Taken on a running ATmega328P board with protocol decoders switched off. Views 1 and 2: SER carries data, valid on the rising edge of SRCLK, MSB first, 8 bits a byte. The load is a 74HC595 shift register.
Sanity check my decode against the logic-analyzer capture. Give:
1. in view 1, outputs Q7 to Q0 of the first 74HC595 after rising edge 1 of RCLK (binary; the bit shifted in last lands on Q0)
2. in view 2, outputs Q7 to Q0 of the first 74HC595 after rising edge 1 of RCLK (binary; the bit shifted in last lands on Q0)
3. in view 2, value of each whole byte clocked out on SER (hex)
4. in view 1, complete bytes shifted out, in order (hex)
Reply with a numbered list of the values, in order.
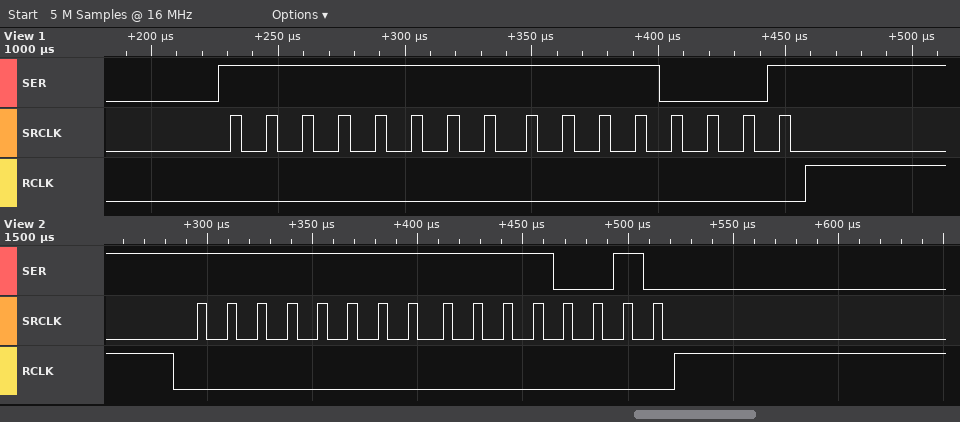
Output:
1. 11110001
2. 11110010
3. 0xFF 0xF2
4. FF F1
